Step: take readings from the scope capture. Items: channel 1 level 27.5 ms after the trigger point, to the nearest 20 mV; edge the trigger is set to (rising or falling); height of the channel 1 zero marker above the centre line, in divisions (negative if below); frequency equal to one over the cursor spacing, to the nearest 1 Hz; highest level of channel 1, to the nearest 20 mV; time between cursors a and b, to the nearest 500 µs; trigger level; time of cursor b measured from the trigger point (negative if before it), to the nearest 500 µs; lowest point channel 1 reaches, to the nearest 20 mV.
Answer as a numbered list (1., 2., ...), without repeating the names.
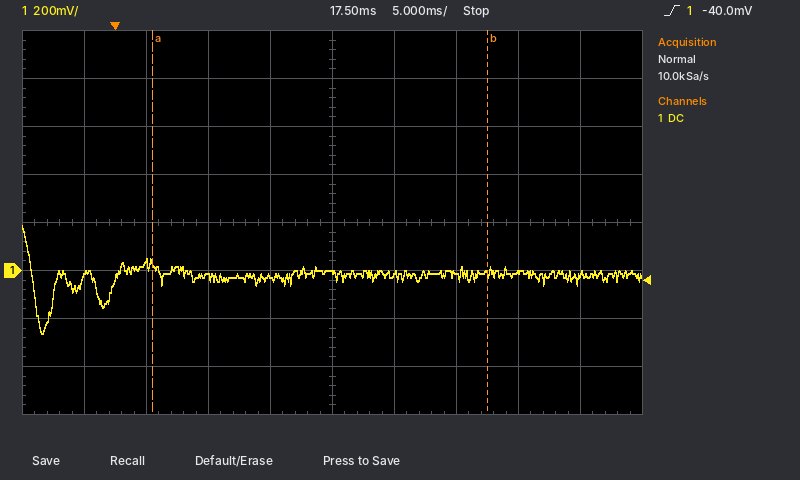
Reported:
1. -20 mV
2. rising
3. -1.0 div
4. 37 Hz
5. 180 mV
6. 27.0 ms
7. -40.0 mV
8. +30.0 ms
9. -260 mV
